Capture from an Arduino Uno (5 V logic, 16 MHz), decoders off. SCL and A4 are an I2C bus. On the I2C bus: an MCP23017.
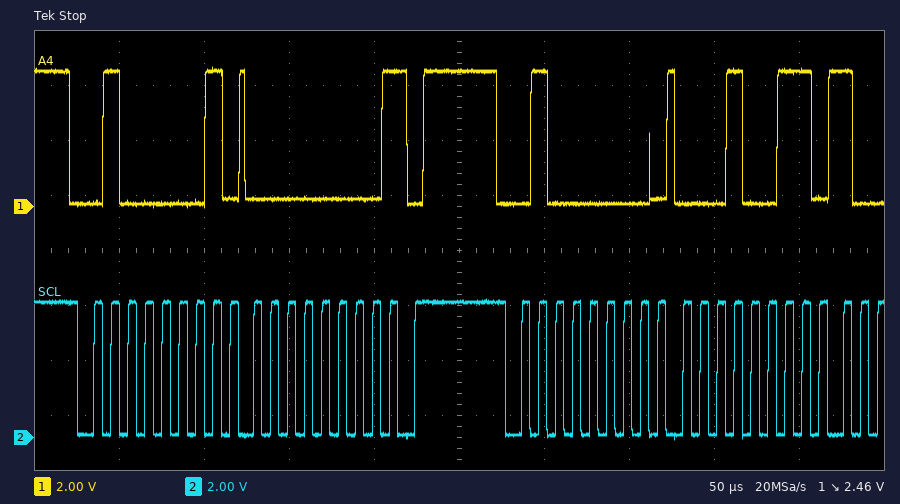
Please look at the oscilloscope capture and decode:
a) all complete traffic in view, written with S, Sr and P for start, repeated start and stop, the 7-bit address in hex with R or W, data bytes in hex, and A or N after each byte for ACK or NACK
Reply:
S 20R A 00 N P S 20W A 13 A
